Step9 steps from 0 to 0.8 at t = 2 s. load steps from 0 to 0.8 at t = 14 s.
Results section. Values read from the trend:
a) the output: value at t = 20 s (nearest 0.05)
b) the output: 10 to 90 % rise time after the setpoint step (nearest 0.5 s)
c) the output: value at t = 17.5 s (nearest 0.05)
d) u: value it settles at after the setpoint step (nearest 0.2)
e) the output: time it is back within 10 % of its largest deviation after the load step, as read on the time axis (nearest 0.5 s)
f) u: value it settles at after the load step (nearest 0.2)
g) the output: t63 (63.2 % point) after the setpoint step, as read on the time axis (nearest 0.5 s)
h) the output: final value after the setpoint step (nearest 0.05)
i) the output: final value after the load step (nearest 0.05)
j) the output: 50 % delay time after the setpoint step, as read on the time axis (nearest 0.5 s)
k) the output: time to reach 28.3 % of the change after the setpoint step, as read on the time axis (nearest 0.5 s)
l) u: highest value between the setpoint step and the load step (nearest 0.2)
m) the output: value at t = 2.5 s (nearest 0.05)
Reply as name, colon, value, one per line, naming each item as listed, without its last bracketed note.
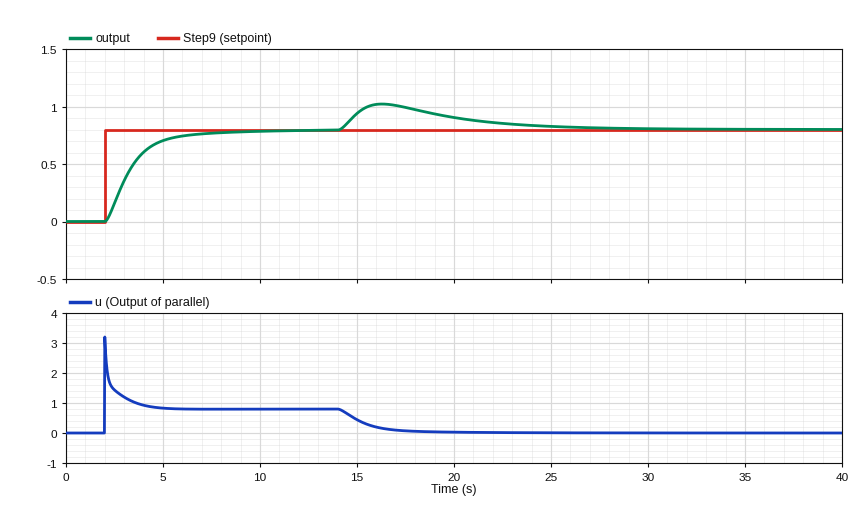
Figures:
the output: value at t = 20 s: 0.90
the output: 10 to 90 % rise time after the setpoint step: 3.0 s
the output: value at t = 17.5 s: 1.00
u: value it settles at after the setpoint step: 0.8
the output: time it is back within 10 % of its largest deviation after the load step, as read on the time axis: 25.5 s
u: value it settles at after the load step: 0.0
the output: t63 (63.2 % point) after the setpoint step, as read on the time axis: 3.5 s
the output: final value after the setpoint step: 0.80
the output: final value after the load step: 0.80
the output: 50 % delay time after the setpoint step, as read on the time axis: 3.0 s
the output: time to reach 28.3 % of the change after the setpoint step, as read on the time axis: 2.5 s
u: highest value between the setpoint step and the load step: 3.2
the output: value at t = 2.5 s: 0.15
